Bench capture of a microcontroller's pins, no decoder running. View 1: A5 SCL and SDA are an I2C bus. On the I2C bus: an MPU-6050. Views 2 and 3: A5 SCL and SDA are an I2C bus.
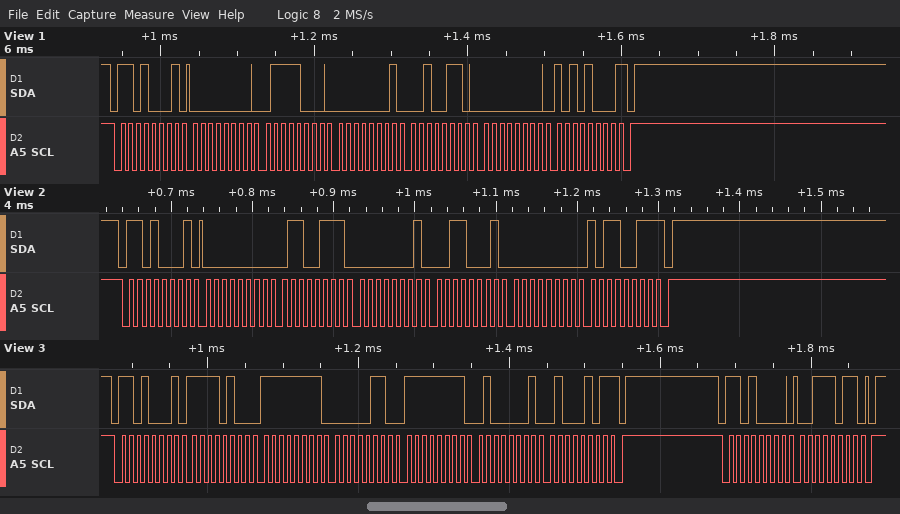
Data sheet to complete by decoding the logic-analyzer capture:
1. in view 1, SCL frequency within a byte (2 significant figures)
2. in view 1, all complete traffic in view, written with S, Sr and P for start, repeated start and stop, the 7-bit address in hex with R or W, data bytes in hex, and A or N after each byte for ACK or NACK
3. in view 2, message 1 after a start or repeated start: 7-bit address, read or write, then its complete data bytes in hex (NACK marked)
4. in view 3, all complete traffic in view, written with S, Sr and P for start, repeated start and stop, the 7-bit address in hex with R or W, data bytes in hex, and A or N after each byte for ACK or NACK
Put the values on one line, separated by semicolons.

100 kHz; S 68R A 00 A 78 A 01 A 26 A 00 A A8 N P; 0x68 read: 00 67 01 31 00 B3 NACK; S 68R A F4 A FF A 06 A FF A 41 A 45 N P S 68W A 3B A P
